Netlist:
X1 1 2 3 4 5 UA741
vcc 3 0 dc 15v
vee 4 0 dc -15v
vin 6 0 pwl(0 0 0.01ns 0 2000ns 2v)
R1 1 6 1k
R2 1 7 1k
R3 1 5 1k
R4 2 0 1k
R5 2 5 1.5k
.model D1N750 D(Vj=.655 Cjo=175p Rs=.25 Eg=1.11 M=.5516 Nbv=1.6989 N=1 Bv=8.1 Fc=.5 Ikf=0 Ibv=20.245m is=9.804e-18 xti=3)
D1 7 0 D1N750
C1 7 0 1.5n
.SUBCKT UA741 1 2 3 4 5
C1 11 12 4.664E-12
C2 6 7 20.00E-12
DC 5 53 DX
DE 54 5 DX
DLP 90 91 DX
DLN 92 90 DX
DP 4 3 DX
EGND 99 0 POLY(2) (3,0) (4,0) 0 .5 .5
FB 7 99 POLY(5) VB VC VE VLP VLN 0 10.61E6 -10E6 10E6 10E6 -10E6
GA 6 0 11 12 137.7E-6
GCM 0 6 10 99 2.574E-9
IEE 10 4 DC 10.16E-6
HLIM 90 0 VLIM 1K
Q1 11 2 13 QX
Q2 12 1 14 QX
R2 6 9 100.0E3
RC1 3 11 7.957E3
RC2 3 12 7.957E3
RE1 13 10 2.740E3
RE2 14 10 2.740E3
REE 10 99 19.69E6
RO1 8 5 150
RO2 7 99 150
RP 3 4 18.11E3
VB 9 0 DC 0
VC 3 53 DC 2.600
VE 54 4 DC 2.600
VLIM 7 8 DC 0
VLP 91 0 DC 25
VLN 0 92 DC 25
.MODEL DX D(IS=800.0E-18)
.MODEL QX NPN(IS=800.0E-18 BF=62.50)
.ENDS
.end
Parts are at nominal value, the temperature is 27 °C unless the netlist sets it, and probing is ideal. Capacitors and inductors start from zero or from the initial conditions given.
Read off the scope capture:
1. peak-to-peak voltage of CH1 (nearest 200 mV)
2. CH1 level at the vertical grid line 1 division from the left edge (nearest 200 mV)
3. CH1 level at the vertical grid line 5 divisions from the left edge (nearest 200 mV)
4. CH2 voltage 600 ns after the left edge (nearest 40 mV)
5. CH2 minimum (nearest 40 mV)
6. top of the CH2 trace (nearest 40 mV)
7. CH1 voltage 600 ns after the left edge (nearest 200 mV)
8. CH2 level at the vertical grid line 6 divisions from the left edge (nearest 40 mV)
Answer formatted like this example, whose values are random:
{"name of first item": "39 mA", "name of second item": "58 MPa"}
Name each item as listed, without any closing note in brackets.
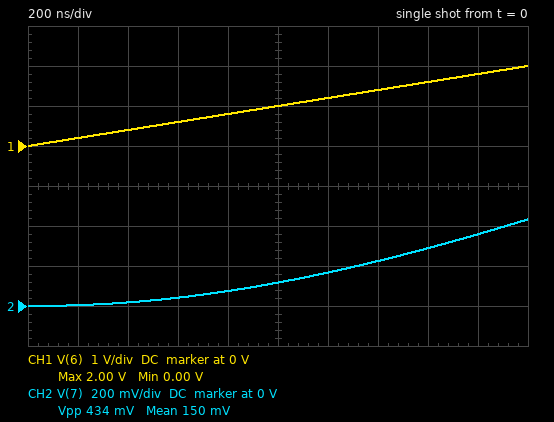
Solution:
{"peak-to-peak voltage of CH1": "2.0 V", "CH1 level at the vertical grid line 1 division from the left edge": "200 mV", "CH1 level at the vertical grid line 5 divisions from the left edge": "1.0 V", "CH2 voltage 600 ns after the left edge": "40 mV", "CH2 minimum": "0 V", "top of the CH2 trace": "440 mV", "CH1 voltage 600 ns after the left edge": "600 mV", "CH2 level at the vertical grid line 6 divisions from the left edge": "160 mV"}
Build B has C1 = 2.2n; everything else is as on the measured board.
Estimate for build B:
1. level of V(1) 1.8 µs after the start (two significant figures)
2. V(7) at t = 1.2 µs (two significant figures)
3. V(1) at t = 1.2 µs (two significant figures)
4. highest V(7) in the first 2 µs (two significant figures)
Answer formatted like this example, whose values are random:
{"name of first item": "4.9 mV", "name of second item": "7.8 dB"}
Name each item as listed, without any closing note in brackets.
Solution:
{"level of V(1) 1.8 µs after the start": "970 mV", "V(7) at t = 1.2 µs": "120 mV", "V(1) at t = 1.2 µs": "610 mV", "highest V(7) in the first 2 µs": "330 mV"}
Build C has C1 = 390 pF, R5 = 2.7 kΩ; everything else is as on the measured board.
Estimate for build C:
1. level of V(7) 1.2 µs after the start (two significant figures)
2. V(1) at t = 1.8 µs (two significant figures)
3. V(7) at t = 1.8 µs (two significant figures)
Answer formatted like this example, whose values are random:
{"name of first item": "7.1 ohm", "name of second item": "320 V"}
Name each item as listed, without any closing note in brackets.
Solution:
{"level of V(7) 1.2 µs after the start": "370 mV", "V(1) at t = 1.8 µs": "1.1 V", "V(7) at t = 1.8 µs": "690 mV"}
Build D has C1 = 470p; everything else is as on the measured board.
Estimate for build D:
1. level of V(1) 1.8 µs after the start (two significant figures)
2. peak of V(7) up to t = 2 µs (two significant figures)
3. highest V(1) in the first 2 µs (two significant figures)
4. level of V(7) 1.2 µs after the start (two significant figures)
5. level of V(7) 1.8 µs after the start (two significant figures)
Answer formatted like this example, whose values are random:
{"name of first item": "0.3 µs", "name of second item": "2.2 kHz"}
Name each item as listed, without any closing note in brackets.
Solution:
{"level of V(1) 1.8 µs after the start": "1.1 V", "peak of V(7) up to t = 2 µs": "750 mV", "highest V(1) in the first 2 µs": "1.2 V", "level of V(7) 1.2 µs after the start": "340 mV", "level of V(7) 1.8 µs after the start": "640 mV"}
